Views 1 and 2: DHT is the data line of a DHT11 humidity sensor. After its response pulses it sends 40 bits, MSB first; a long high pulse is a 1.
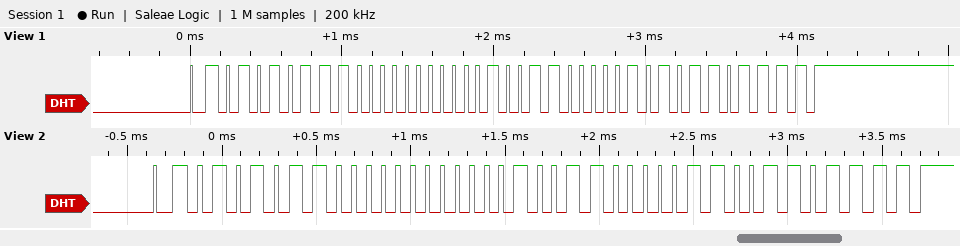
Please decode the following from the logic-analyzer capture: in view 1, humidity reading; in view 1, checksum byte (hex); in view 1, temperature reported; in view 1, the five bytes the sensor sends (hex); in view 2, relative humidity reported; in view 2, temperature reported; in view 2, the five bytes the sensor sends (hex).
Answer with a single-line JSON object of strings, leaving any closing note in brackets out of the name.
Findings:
{"in view 1, humidity reading": "87 %", "in view 1, checksum byte": "0x6F", "in view 1, temperature reported": "19.5 °C", "in view 1, the five bytes the sensor sends": "57 00 13 05 6F", "in view 2, relative humidity reported": "86 %", "in view 2, temperature reported": "19.6 °C", "in view 2, the five bytes the sensor sends": "56 00 13 06 6F"}
